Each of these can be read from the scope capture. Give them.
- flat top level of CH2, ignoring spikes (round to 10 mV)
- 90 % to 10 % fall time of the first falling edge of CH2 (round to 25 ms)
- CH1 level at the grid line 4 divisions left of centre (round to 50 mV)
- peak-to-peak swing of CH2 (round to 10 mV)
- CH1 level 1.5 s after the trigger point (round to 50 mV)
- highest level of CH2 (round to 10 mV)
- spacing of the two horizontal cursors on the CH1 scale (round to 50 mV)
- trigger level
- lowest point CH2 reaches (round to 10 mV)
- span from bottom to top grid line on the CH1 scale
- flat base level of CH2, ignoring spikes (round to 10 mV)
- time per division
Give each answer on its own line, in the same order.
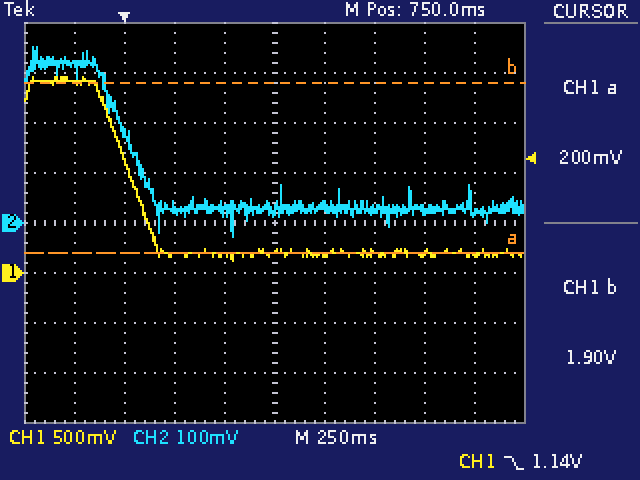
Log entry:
320 mV
250 ms
1.90 V
380 mV
200 mV
350 mV
1.70 V
1.14 V
-30 mV
4 V
30 mV
250 ms
